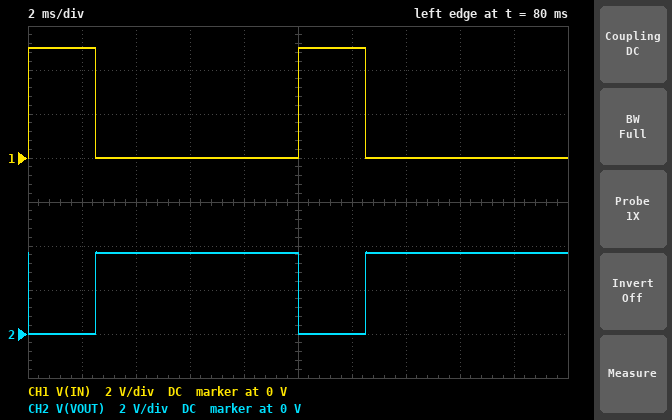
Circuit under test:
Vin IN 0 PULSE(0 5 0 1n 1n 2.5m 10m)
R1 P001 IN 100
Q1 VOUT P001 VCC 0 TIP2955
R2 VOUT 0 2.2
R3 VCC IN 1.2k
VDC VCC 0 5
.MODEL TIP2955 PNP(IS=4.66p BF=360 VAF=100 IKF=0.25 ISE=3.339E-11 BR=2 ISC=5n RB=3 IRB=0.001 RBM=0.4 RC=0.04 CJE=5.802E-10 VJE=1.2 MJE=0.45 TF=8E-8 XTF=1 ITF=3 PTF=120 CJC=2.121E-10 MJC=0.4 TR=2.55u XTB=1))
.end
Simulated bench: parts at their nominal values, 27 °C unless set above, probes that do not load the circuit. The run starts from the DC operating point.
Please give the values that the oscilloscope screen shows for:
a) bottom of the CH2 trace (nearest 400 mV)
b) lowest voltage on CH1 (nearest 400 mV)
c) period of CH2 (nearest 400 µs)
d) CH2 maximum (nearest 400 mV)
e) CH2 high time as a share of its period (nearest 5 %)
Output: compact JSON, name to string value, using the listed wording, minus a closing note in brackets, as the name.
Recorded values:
{"bottom of the CH2 trace": "0 V", "lowest voltage on CH1": "0 V", "period of CH2": "10.0 ms", "CH2 maximum": "3.6 V", "CH2 high time as a share of its period": "75 %"}
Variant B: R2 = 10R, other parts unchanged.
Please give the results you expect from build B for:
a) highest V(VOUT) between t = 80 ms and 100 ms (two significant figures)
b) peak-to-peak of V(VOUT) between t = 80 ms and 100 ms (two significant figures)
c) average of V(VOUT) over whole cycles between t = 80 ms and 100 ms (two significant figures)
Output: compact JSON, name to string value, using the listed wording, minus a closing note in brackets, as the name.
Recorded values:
{"highest V(VOUT) between t = 80 ms and 100 ms": "4.9 V", "peak-to-peak of V(VOUT) between t = 80 ms and 100 ms": "5.0 V", "average of V(VOUT) over whole cycles between t = 80 ms and 100 ms": "3.7 V"}
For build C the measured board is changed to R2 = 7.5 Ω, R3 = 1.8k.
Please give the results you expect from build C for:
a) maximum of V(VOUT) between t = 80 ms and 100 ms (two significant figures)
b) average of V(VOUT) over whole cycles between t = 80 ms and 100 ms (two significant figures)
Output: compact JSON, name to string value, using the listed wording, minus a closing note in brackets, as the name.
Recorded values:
{"maximum of V(VOUT) between t = 80 ms and 100 ms": "4.9 V", "average of V(VOUT) over whole cycles between t = 80 ms and 100 ms": "3.7 V"}
